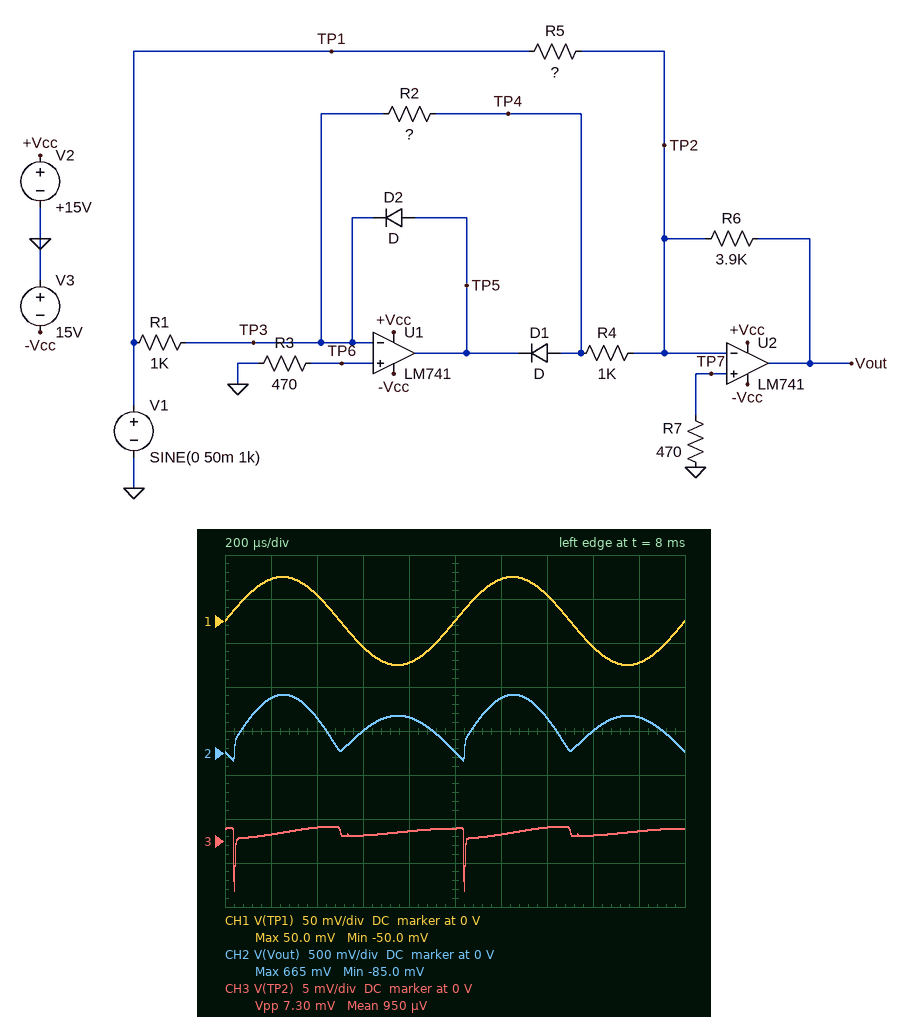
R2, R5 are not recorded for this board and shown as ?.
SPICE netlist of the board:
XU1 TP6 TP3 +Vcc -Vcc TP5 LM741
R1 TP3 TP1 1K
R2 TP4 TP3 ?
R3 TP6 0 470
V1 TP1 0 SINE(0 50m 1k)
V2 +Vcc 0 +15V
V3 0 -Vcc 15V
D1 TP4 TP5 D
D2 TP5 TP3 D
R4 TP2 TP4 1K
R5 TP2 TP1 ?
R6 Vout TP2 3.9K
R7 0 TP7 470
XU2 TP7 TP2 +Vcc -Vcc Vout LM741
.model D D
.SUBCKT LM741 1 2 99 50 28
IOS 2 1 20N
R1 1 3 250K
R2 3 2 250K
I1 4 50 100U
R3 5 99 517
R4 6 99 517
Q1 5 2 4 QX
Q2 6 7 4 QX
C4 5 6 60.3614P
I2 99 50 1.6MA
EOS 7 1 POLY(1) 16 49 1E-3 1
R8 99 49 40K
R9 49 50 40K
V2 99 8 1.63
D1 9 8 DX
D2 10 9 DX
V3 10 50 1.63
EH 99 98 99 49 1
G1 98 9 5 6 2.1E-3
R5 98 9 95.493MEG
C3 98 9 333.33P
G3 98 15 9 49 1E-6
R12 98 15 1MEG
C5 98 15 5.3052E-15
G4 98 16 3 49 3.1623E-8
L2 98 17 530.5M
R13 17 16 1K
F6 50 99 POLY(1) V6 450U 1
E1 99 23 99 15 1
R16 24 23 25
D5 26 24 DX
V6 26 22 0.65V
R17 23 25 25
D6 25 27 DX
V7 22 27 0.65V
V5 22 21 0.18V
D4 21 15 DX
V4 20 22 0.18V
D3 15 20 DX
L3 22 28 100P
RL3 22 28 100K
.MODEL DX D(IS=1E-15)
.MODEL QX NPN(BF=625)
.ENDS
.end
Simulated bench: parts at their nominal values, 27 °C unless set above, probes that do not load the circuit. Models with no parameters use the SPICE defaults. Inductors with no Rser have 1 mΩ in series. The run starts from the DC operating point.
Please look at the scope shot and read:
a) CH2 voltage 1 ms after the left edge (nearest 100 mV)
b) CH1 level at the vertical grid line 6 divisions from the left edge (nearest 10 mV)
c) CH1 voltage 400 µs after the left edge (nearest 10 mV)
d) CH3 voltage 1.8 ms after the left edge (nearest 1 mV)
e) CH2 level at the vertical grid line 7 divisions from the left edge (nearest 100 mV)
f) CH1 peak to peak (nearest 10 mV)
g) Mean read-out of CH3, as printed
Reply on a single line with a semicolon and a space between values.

0 V; 50 mV; 30 mV; 1 mV; 400 mV; 100 mV; 950 µV
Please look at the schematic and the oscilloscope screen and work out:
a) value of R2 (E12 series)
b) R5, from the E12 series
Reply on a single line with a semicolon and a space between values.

5.6 kΩ; 470 Ω
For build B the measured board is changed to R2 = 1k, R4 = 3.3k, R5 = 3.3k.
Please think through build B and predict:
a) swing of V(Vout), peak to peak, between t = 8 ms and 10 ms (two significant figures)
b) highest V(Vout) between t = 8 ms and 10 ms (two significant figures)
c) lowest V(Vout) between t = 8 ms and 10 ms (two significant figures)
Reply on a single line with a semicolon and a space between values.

80 mV; 62 mV; -18 mV
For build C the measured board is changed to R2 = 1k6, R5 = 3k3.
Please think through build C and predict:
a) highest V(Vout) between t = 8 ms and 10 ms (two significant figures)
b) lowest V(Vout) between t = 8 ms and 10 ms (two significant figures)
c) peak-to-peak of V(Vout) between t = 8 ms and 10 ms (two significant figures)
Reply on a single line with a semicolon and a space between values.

250 mV; -23 mV; 270 mV
